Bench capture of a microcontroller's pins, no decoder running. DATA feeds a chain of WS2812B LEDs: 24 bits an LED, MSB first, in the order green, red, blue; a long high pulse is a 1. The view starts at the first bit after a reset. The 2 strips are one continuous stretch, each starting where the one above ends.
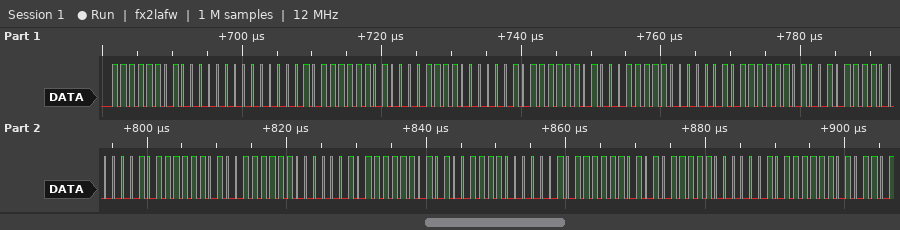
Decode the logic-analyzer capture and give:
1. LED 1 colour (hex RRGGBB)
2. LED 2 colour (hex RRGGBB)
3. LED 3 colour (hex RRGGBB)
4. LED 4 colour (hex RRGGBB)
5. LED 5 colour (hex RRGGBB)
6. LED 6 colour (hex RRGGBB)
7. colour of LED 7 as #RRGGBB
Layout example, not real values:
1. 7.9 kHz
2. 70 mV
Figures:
1. #00FD02
2. #0FFD02
3. #1FFD02
4. #2FFD02
5. #3FFD02
6. #4FFD02
7. #5FFD02
